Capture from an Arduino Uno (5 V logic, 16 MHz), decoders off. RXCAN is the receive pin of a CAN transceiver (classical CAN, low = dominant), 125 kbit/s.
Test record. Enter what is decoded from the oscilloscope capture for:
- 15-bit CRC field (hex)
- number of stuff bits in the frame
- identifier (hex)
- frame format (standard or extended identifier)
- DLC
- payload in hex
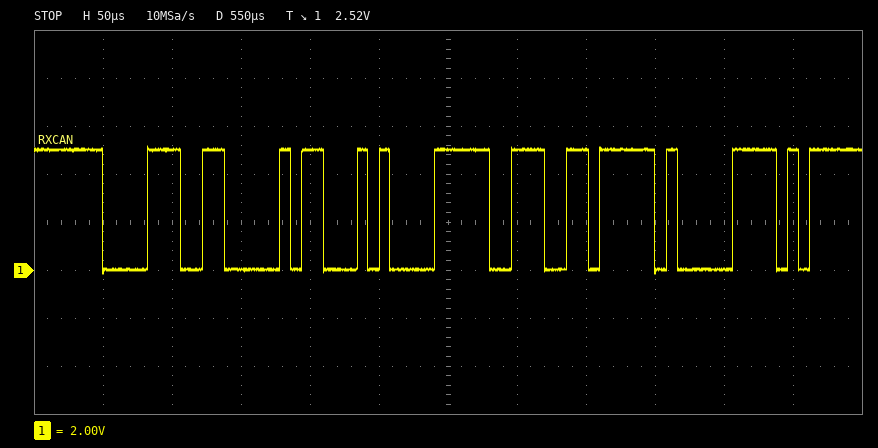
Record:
0x7E0E
4
0x0E6
standard
3
14 3E E6
